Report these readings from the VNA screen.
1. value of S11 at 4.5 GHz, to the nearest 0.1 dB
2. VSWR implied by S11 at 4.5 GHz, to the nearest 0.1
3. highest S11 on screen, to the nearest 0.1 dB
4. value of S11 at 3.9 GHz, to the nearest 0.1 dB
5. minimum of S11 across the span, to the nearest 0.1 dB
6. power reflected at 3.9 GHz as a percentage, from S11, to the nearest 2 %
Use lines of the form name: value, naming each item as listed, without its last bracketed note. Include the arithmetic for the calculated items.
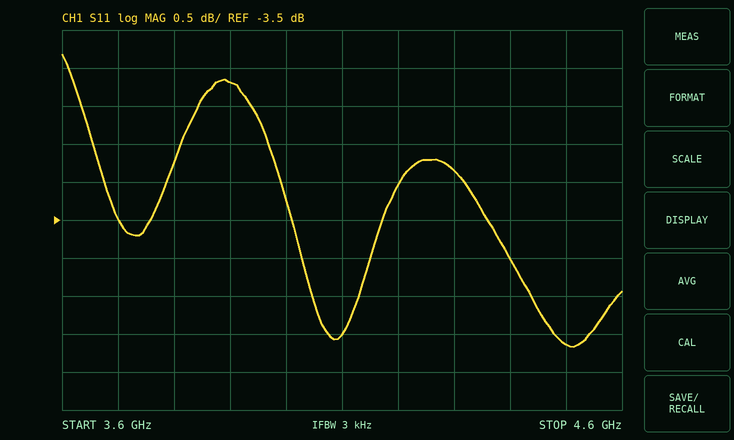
value of S11 at 4.5 GHz, to the nearest 0.1 dB: -5.1 dB
VSWR implied by S11 at 4.5 GHz, to the nearest 0.1: |Γ| = 10^(-5.1/20) = 0.5559; VSWR = (1 + 0.5559)/(1 − 0.5559) ≈ 3.5
highest S11 on screen, to the nearest 0.1 dB: -1.3 dB
value of S11 at 3.9 GHz, to the nearest 0.1 dB: -1.7 dB
minimum of S11 across the span, to the nearest 0.1 dB: -5.2 dB
power reflected at 3.9 GHz as a percentage, from S11, to the nearest 2 %: 10^(-1.7/10) ≈ 68 %
